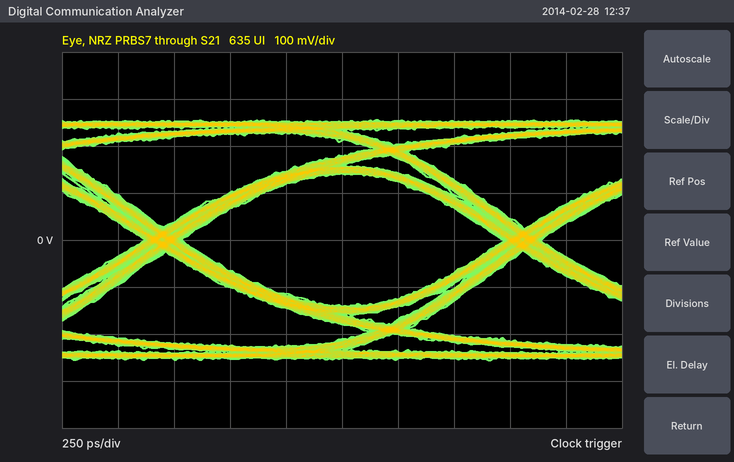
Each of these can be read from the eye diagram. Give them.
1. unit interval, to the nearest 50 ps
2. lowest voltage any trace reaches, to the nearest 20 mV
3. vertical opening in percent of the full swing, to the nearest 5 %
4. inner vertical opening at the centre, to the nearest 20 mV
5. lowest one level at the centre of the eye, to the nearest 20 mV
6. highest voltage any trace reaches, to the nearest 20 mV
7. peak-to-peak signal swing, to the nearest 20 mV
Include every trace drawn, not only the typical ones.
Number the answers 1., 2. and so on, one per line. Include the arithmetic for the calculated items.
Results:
1. 1.60 ns
2. -260 mV
3. 280 mV / 520 mV ≈ 53.8 %, so 55 % to the nearest 5 %
4. 280 mV
5. 140 mV
6. 260 mV
7. 520 mV
